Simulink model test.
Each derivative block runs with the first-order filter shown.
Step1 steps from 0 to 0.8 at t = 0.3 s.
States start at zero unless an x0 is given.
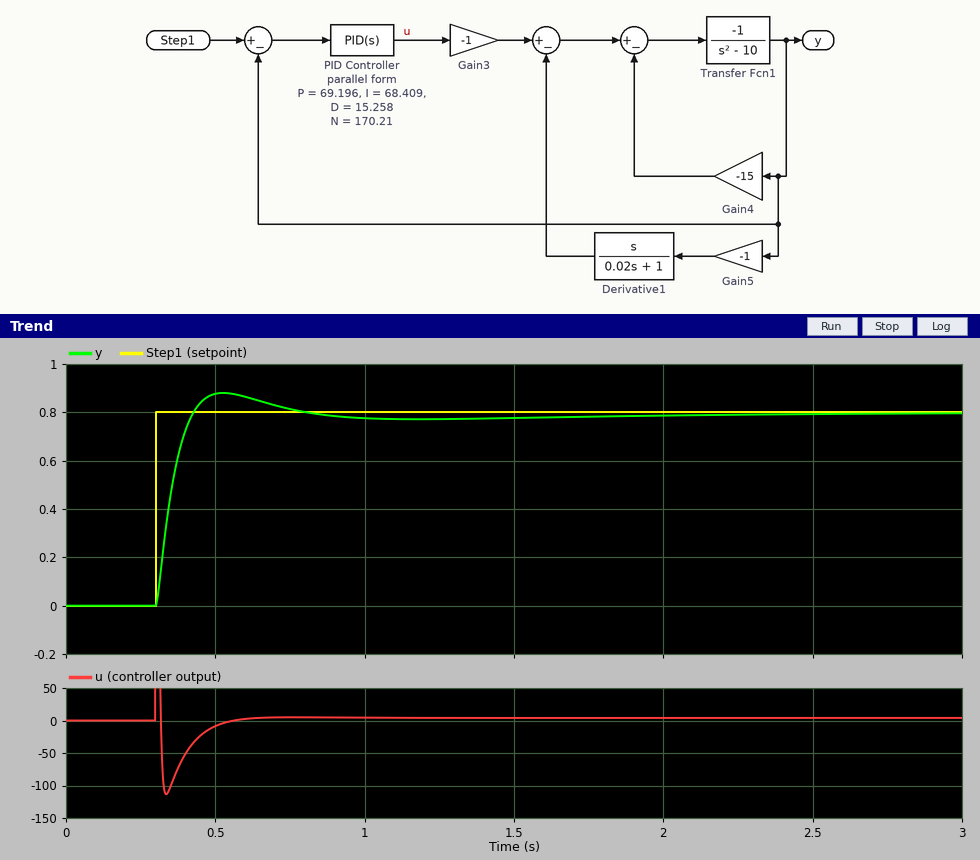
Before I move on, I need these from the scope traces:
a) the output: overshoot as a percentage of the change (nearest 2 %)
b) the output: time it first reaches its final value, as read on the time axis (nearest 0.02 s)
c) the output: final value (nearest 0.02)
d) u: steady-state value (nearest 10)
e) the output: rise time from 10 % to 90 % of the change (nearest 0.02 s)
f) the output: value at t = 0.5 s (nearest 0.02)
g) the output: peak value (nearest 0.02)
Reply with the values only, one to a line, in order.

10 %
0.42 s
0.80
0
0.08 s
0.88
0.88
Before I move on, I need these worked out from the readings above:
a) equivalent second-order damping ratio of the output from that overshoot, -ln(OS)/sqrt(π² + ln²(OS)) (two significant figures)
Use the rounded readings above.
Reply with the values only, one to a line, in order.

0.59
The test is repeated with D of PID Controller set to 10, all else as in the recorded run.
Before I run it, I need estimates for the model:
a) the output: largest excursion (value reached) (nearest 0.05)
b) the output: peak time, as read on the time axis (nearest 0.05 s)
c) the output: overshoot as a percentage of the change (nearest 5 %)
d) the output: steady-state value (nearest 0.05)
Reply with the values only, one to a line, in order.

0.95
0.55 s
20 %
0.80
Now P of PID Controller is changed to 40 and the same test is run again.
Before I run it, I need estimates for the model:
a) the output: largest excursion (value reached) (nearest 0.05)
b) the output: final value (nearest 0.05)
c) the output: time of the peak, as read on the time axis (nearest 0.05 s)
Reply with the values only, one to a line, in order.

0.85
0.80
0.55 s
